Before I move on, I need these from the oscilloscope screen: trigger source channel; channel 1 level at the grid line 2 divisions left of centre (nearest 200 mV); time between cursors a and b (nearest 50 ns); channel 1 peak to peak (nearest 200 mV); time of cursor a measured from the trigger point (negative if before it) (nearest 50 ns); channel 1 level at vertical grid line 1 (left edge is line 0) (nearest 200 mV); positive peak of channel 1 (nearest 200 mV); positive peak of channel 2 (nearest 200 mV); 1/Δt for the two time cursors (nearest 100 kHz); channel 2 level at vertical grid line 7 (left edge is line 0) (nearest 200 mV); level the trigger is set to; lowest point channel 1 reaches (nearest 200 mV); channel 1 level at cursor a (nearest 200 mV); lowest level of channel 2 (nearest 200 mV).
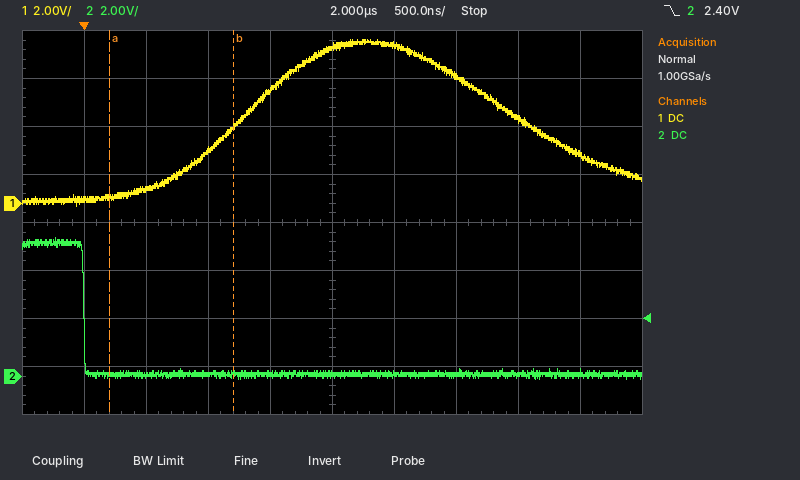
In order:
channel 2
2.2 V
1.00 µs
7.0 V
+200 ns
200 mV
6.8 V
5.8 V
1.0 MHz
0.0 V
2.40 V
-200 mV
200 mV
-200 mV
